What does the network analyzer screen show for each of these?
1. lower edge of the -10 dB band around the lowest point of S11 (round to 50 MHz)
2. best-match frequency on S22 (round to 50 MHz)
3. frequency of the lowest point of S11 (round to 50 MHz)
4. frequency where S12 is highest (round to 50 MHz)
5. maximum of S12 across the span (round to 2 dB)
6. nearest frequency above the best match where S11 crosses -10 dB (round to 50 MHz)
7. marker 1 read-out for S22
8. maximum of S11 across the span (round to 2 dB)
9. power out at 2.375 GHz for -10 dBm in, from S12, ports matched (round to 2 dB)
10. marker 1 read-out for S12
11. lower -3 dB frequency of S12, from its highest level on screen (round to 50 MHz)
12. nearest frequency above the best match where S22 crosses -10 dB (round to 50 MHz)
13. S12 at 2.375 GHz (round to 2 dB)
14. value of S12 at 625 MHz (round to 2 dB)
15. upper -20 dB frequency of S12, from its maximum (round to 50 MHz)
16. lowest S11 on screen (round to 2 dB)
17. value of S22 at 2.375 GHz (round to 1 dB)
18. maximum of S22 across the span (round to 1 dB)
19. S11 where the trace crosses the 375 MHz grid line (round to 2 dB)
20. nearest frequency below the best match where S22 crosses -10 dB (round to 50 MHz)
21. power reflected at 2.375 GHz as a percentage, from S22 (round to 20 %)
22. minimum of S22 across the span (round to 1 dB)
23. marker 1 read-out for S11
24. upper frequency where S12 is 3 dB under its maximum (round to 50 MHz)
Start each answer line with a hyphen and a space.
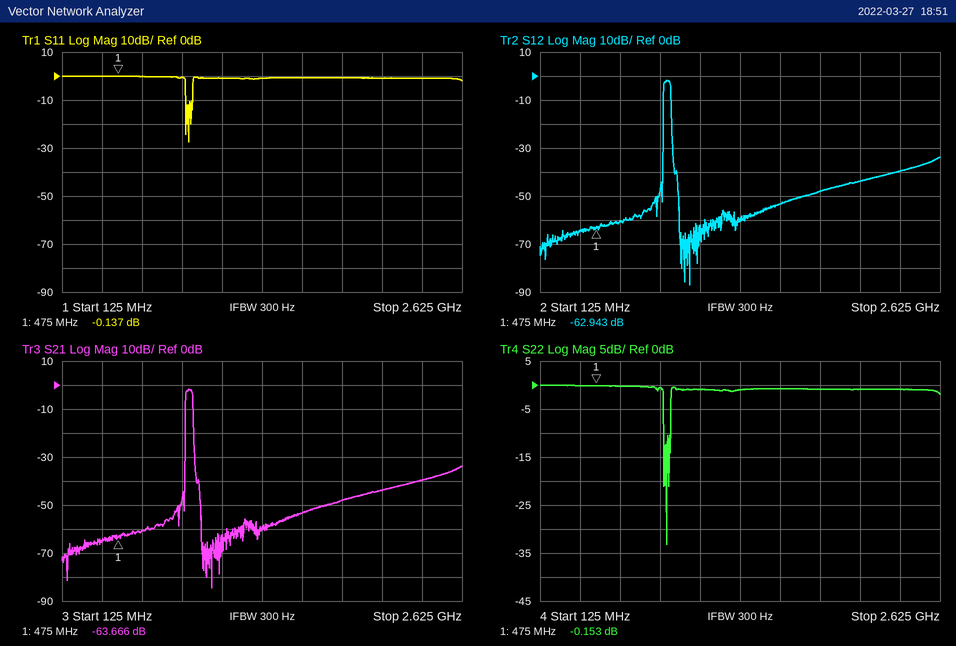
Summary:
- 900 MHz
- 900 MHz
- 900 MHz
- 900 MHz
- -2 dB
- 950 MHz
- -0.153 dB
- 0 dB
- -50 dBm
- -62.943 dB
- 900 MHz
- 950 MHz
- -40 dB
- -60 dB
- 950 MHz
- -28 dB
- -1 dB
- 0 dB
- 0 dB
- 900 MHz
- 80 %
- -33 dB
- -0.137 dB
- 950 MHz
